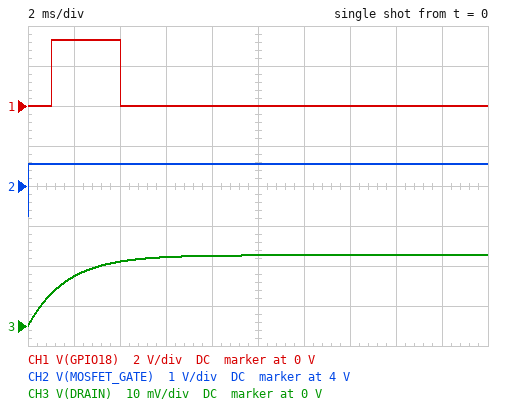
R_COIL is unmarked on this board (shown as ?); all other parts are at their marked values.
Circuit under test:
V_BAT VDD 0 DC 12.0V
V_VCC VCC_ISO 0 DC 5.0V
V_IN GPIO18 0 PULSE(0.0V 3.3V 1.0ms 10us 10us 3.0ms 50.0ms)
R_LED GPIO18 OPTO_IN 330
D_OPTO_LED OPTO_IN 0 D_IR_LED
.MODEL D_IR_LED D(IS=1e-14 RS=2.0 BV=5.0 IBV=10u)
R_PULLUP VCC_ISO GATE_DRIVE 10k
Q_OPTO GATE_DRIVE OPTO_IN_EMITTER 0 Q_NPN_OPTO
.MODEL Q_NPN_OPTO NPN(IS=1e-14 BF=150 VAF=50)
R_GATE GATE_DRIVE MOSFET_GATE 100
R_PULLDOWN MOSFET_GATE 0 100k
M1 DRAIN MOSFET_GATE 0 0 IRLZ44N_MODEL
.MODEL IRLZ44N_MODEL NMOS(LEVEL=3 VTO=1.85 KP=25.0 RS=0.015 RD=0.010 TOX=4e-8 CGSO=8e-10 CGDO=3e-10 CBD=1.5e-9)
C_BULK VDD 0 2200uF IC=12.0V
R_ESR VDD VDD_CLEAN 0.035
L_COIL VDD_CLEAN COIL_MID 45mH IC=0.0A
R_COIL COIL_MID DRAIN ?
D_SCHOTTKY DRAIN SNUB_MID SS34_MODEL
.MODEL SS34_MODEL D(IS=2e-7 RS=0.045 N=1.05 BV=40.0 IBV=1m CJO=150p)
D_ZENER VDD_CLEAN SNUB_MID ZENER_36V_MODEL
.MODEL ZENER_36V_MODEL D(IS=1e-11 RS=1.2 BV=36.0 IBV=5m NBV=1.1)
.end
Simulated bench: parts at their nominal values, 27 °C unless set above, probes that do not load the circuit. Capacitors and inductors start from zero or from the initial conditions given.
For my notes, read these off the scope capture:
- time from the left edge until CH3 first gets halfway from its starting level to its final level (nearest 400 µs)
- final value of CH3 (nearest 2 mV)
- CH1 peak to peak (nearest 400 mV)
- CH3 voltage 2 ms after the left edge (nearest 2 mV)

1.2 ms
18 mV
3.2 V
12 mV
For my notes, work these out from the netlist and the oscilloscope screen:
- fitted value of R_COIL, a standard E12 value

27 Ω
